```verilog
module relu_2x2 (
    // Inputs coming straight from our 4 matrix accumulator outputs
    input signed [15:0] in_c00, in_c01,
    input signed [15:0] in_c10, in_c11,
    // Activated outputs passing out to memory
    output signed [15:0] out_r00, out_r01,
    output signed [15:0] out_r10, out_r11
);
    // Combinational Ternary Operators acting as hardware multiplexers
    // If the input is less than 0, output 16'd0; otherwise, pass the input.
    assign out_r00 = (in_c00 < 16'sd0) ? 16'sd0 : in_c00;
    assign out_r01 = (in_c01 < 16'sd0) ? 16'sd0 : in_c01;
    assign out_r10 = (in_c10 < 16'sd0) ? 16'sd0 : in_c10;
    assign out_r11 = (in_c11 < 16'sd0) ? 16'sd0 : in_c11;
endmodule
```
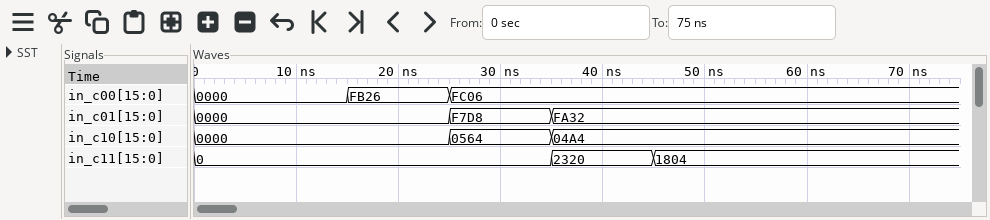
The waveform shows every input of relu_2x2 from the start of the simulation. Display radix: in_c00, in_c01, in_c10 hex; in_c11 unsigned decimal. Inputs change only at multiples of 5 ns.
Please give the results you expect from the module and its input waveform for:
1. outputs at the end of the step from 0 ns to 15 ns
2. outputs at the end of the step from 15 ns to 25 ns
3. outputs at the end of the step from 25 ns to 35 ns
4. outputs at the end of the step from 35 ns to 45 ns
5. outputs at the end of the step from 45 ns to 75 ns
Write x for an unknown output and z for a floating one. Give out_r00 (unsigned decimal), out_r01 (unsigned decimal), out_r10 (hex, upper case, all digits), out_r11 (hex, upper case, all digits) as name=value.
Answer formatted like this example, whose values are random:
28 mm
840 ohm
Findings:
out_r00=0, out_r01=0, out_r10=0000, out_r11=0000
out_r00=0, out_r01=0, out_r10=0000, out_r11=0000
out_r00=0, out_r01=0, out_r10=0564, out_r11=0000
out_r00=0, out_r01=0, out_r10=04A4, out_r11=0910
out_r00=0, out_r01=0, out_r10=04A4, out_r11=070C
